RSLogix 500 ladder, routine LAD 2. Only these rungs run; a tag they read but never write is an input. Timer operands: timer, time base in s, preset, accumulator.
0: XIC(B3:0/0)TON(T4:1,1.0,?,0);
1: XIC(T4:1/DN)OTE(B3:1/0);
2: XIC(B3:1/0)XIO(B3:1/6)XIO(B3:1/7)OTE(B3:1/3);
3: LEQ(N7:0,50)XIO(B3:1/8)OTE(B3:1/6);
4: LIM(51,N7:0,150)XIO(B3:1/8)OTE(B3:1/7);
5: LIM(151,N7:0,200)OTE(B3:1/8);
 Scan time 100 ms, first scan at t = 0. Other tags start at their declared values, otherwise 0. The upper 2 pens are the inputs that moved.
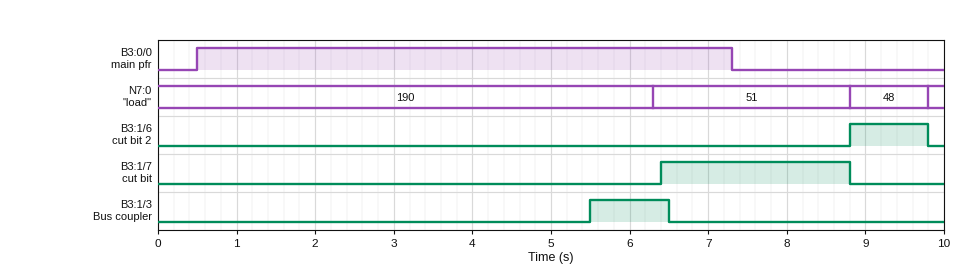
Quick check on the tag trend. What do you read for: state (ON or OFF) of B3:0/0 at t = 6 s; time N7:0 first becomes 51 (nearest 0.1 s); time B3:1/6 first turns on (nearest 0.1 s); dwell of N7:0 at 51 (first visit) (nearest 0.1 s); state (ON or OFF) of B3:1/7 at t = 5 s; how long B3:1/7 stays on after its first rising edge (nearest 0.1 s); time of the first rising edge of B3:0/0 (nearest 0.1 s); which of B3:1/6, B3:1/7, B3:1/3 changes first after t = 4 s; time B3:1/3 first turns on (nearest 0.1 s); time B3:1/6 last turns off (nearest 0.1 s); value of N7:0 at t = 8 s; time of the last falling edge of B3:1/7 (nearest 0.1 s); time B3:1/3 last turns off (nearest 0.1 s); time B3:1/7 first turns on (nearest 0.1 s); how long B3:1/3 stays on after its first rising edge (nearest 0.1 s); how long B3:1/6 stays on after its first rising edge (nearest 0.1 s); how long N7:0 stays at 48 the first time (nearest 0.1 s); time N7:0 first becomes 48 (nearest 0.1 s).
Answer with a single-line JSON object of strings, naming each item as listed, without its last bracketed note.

{"state (ON or OFF) of B3:0/0 at t = 6 s": "ON", "time N7:0 first becomes 51": "6.3 s", "time B3:1/6 first turns on": "8.8 s", "dwell of N7:0 at 51 (first visit)": "2.5 s", "state (ON or OFF) of B3:1/7 at t = 5 s": "OFF", "how long B3:1/7 stays on after its first rising edge": "2.4 s", "time of the first rising edge of B3:0/0": "0.5 s", "which of B3:1/6, B3:1/7, B3:1/3 changes first after t = 4 s": "B3:1/3", "time B3:1/3 first turns on": "5.5 s", "time B3:1/6 last turns off": "9.8 s", "value of N7:0 at t = 8 s": "51", "time of the last falling edge of B3:1/7": "8.8 s", "time B3:1/3 last turns off": "6.5 s", "time B3:1/7 first turns on": "6.4 s", "how long B3:1/3 stays on after its first rising edge": "1.0 s", "how long B3:1/6 stays on after its first rising edge": "1.0 s", "how long N7:0 stays at 48 the first time": "1.0 s", "time N7:0 first becomes 48": "8.8 s"}
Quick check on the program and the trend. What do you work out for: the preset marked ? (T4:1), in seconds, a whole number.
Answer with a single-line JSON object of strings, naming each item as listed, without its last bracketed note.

{"the preset marked ? (T4:1), in seconds, a whole number": "5 s"}
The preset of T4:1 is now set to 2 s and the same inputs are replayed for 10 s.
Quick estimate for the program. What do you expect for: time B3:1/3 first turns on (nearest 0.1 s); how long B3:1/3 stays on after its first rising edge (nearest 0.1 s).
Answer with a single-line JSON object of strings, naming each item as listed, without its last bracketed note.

{"time B3:1/3 first turns on": "2.5 s", "how long B3:1/3 stays on after its first rising edge": "4.0 s"}
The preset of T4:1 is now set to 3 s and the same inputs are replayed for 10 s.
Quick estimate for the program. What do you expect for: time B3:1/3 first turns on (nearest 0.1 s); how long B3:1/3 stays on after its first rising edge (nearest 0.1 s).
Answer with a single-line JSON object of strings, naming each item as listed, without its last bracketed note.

{"time B3:1/3 first turns on": "3.5 s", "how long B3:1/3 stays on after its first rising edge": "3.0 s"}
